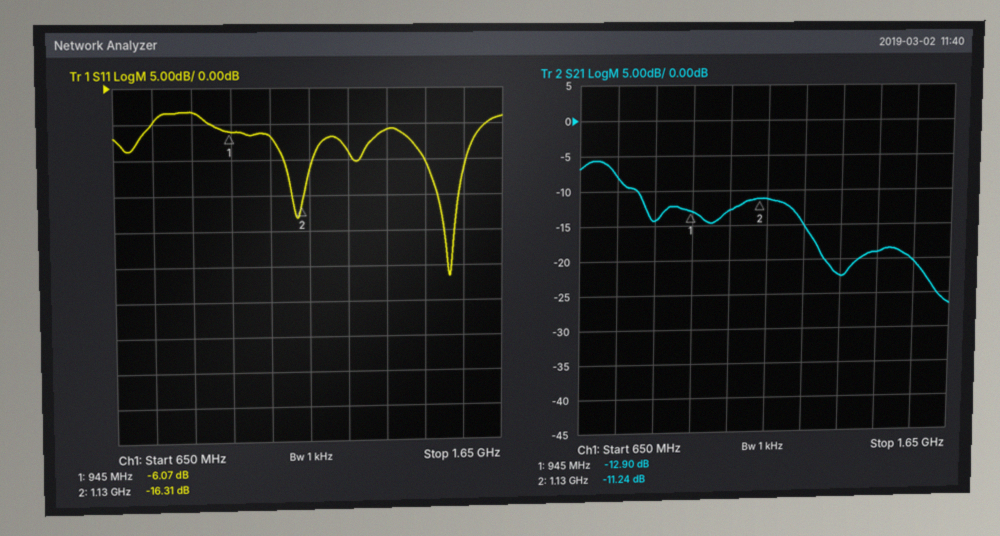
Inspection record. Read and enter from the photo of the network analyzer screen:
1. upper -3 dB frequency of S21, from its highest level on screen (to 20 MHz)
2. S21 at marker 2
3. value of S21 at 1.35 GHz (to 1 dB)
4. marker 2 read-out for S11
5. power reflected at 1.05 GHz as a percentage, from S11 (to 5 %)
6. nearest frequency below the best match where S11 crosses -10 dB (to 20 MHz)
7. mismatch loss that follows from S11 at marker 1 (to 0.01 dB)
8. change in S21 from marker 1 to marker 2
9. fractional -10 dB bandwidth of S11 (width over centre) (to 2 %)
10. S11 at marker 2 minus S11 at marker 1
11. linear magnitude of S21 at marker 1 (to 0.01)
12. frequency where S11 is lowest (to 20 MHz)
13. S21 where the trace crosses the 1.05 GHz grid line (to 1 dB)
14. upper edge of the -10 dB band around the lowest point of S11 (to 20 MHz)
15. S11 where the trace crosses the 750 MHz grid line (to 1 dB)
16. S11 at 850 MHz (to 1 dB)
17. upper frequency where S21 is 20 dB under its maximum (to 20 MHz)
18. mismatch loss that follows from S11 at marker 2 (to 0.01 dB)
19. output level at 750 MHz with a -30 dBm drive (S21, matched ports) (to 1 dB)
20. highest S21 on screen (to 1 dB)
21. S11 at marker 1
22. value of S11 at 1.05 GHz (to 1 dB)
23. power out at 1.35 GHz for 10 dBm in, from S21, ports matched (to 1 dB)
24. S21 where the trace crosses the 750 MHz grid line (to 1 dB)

760 MHz
-11.24 dB
-22 dB
-16.31 dB
20 %
1.44 GHz
1.23 dB
1.66 dB
8 %
-10.24 dB
0.23
1.52 GHz
-13 dB
1.56 GHz
-5 dB
-3 dB
1.62 GHz
0.10 dB
-38 dBm
-6 dB
-6.07 dB
-7 dB
-12 dBm
-8 dB
